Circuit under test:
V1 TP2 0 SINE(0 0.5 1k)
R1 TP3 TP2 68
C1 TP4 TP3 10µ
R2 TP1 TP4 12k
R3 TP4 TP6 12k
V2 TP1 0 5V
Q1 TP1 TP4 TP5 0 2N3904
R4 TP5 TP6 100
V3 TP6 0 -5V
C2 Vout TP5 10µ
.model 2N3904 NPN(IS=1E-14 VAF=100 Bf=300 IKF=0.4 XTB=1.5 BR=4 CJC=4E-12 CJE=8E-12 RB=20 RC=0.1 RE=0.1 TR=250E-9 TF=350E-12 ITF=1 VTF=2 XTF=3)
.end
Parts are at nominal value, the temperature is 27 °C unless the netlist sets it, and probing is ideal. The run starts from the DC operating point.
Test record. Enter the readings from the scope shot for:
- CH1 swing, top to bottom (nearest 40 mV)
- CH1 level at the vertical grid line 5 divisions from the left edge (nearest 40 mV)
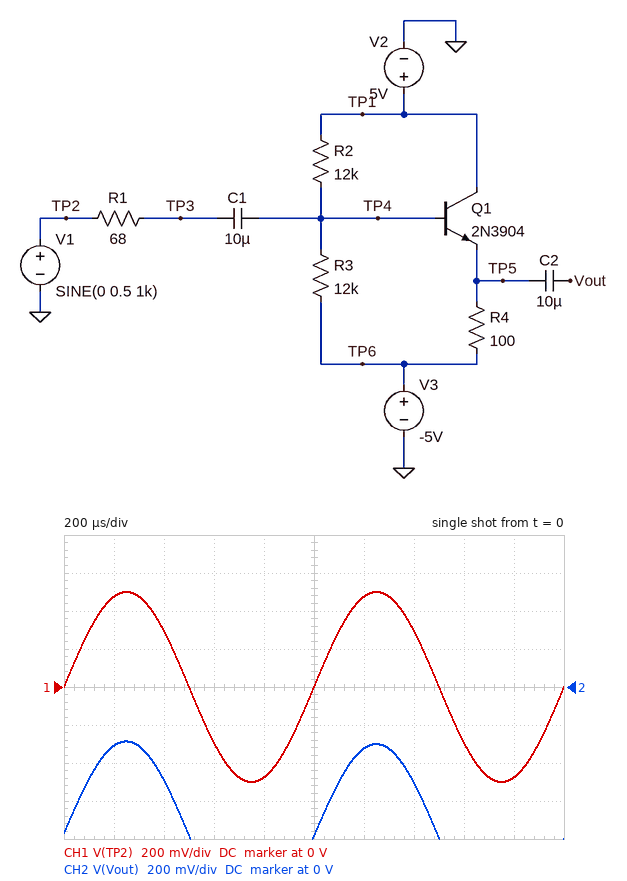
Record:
1.00 V
0 V
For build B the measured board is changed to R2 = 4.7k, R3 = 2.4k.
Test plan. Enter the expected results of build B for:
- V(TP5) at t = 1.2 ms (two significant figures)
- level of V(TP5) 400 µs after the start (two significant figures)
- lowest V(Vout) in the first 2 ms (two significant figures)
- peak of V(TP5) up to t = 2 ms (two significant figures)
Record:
-510 mV
-610 mV
-1.5 V
-390 mV
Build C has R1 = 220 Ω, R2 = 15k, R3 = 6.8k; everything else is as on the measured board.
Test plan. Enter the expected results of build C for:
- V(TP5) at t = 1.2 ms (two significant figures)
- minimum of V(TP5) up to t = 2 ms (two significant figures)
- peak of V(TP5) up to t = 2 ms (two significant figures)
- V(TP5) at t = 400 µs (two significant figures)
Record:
-490 mV
-1.4 V
-420 mV
-620 mV
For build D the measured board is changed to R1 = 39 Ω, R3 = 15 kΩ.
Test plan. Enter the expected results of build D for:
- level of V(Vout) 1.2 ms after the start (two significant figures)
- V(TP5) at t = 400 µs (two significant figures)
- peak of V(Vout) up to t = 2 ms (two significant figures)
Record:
-300 mV
-480 mV
-270 mV
